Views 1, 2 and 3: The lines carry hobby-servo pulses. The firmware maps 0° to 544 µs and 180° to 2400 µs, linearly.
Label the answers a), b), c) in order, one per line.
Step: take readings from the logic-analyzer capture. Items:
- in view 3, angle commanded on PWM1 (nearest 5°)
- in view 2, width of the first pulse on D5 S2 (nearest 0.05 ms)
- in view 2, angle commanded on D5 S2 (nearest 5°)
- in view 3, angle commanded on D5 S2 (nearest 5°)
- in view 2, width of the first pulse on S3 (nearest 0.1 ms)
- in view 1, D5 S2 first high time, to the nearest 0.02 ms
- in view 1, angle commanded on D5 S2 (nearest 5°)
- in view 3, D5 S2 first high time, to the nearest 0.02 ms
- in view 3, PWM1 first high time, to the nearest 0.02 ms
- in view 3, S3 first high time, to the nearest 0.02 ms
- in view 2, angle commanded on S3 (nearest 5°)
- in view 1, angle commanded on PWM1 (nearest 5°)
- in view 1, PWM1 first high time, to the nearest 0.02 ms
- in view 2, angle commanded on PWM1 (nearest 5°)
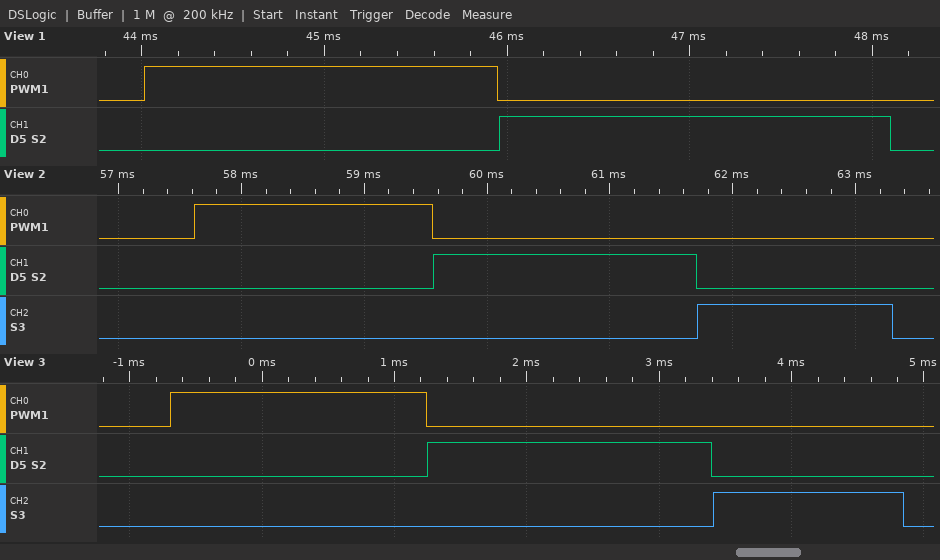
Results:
a) 135°
b) 2.15 ms
c) 155°
d) 155°
e) 1.6 ms
f) 2.14 ms
g) 155°
h) 2.14 ms
i) 1.94 ms
j) 1.44 ms
k) 100°
l) 135°
m) 1.94 ms
n) 135°
